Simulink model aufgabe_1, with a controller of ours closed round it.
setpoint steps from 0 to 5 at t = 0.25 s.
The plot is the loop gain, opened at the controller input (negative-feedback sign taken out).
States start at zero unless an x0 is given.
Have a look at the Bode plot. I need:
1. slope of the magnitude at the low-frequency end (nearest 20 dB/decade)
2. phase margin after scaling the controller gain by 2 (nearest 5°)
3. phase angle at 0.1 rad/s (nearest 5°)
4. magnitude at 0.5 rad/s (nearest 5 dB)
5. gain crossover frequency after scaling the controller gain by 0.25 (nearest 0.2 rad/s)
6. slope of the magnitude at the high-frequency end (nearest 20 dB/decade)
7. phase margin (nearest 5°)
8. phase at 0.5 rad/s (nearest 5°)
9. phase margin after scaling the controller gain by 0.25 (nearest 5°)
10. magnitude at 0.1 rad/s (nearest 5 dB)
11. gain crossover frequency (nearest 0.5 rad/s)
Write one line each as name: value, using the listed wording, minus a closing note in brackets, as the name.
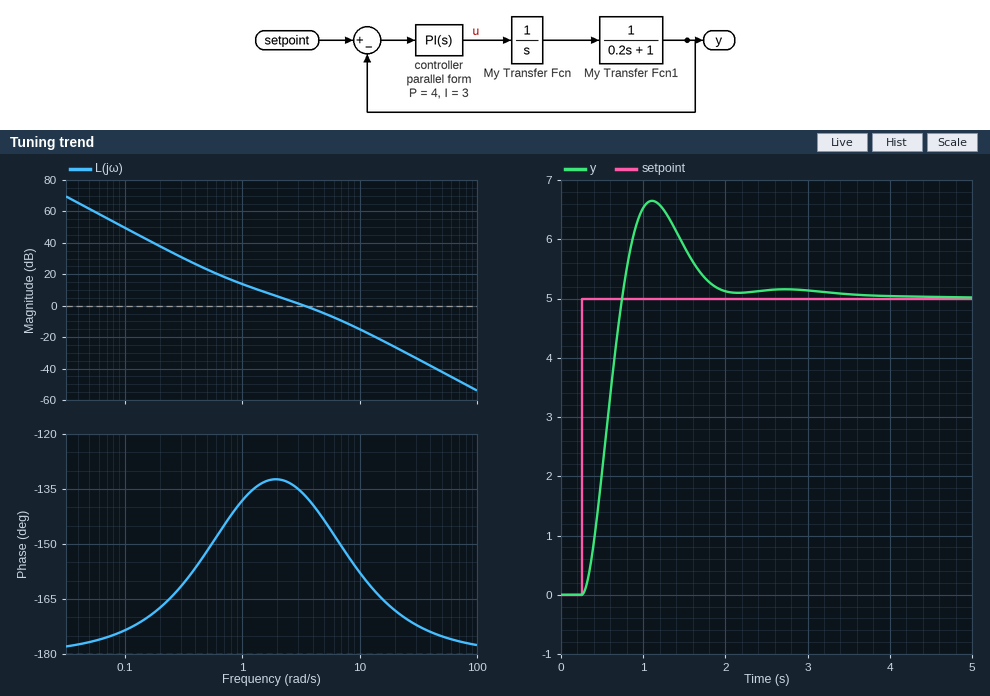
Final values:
slope of the magnitude at the low-frequency end: -40 dB/decade
phase margin after scaling the controller gain by 2: 35°
phase angle at 0.1 rad/s: -175°
magnitude at 0.5 rad/s: 25 dB
gain crossover frequency after scaling the controller gain by 0.25: 1.2 rad/s
slope of the magnitude at the high-frequency end: -40 dB/decade
phase margin: 45°
phase at 0.5 rad/s: -150°
phase margin after scaling the controller gain by 0.25: 45°
magnitude at 0.1 rad/s: 50 dB
gain crossover frequency: 3.5 rad/s
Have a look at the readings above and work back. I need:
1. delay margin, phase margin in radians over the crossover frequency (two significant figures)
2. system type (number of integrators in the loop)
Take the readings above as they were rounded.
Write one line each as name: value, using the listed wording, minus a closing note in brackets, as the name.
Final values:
delay margin, phase margin in radians over the crossover frequency: 0.22 s
system type: 2
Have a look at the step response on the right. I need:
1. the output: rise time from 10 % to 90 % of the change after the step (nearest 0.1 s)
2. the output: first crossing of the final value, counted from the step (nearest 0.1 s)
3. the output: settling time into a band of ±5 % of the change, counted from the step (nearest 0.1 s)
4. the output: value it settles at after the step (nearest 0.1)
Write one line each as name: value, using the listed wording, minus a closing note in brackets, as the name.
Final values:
the output: rise time from 10 % to 90 % of the change after the step: 0.3 s
the output: first crossing of the final value, counted from the step: 0.5 s
the output: settling time into a band of ±5 % of the change, counted from the step: 1.6 s
the output: value it settles at after the step: 5.0
